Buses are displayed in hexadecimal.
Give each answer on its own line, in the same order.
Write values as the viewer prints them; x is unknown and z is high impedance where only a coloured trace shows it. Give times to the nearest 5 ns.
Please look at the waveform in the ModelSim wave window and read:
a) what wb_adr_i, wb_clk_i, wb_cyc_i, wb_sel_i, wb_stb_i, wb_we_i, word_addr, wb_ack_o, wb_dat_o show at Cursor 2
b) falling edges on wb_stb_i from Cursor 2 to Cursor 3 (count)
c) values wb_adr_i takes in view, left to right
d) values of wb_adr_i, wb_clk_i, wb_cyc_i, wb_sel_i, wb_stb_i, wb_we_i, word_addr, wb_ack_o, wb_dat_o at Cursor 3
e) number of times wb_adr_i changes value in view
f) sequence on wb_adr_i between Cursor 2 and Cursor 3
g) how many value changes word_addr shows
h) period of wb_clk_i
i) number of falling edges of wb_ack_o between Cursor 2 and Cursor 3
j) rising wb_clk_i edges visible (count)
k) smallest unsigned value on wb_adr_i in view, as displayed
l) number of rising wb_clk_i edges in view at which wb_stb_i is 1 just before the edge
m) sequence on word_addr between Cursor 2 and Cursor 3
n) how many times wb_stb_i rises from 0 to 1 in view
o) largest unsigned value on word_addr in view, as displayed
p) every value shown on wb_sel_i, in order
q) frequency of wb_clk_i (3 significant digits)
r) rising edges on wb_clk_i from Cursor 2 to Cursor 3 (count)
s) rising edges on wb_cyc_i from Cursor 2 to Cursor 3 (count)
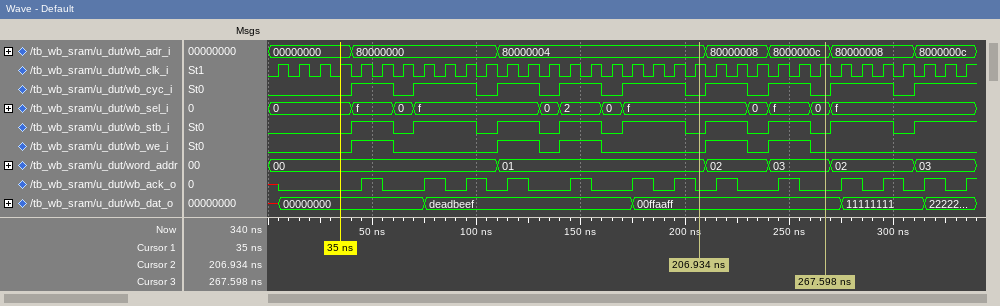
wb_adr_i=80000004, wb_clk_i=1, wb_cyc_i=0, wb_sel_i=f, wb_stb_i=0, wb_we_i=0, word_addr=01, wb_ack_o=0, wb_dat_o=00ffaaff
2
00000000, 80000000, 80000004, 80000008, 8000000c, 80000008, 8000000c
wb_adr_i=8000000c, wb_clk_i=1, wb_cyc_i=0, wb_sel_i=0, wb_stb_i=0, wb_we_i=0, word_addr=03, wb_ack_o=0, wb_dat_o=00ffaaff
6
80000004, 80000008, 8000000c
5
10 ns
2
34
00000000
22
01, 02, 03
9
03
0, f, 0, f, 0, 2, 0, f, 0, f, 0, f
100 MHz
6
2
